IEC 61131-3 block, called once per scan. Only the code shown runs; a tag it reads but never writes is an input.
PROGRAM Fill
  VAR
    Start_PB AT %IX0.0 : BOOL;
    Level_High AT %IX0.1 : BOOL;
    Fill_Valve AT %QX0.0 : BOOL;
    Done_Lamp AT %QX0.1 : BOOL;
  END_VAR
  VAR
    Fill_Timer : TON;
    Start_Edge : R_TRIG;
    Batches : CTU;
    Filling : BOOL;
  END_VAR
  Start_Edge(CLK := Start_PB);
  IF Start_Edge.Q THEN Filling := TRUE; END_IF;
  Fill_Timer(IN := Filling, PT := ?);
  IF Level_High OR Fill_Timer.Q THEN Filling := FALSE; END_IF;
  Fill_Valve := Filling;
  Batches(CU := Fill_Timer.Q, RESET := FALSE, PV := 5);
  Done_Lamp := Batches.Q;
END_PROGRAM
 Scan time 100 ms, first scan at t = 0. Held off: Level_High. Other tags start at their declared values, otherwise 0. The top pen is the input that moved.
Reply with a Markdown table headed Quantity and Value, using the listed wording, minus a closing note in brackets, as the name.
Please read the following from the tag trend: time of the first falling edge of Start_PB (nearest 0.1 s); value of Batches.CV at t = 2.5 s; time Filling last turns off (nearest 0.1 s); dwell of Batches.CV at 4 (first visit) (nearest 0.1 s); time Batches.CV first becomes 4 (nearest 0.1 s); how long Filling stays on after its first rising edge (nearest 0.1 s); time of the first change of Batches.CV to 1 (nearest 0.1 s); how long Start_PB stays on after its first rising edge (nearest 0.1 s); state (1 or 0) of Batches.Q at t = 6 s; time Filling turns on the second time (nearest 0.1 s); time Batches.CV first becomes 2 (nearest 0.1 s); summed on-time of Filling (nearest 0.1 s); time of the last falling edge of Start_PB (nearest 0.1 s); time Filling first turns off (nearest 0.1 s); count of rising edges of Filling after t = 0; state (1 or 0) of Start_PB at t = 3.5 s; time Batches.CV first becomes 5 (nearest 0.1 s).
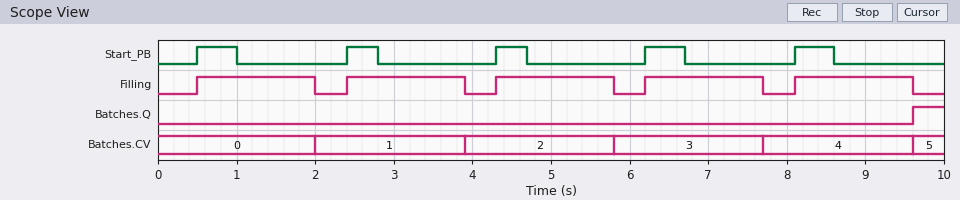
| Quantity | Value |
|---|---|
| time of the first falling edge of Start_PB | 1.0 s |
| value of Batches.CV at t = 2.5 s | 1 |
| time Filling last turns off | 9.6 s |
| dwell of Batches.CV at 4 (first visit) | 1.9 s |
| time Batches.CV first becomes 4 | 7.7 s |
| how long Filling stays on after its first rising edge | 1.5 s |
| time of the first change of Batches.CV to 1 | 2.0 s |
| how long Start_PB stays on after its first rising edge | 0.5 s |
| state (1 or 0) of Batches.Q at t = 6 s | 0 |
| time Filling turns on the second time | 2.4 s |
| time Batches.CV first becomes 2 | 3.9 s |
| summed on-time of Filling | 7.5 s |
| time of the last falling edge of Start_PB | 8.6 s |
| time Filling first turns off | 2.0 s |
| count of rising edges of Filling after t = 0 | 5 |
| state (1 or 0) of Start_PB at t = 3.5 s | 0 |
| time Batches.CV first becomes 5 | 9.6 s |
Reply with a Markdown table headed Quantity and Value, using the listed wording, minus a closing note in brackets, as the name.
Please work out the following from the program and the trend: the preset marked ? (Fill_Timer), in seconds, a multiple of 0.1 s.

| Quantity | Value |
|---|---|
| the preset marked ? (Fill_Timer), in seconds, a multiple of 0.1 s | 1.5 s |
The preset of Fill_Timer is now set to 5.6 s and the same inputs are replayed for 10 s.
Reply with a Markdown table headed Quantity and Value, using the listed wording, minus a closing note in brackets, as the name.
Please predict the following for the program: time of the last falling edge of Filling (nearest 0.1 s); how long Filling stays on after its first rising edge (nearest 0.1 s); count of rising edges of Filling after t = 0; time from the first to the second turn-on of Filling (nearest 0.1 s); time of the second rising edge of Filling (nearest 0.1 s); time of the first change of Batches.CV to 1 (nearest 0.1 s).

| Quantity | Value |
|---|---|
| time of the last falling edge of Filling | 6.1 s |
| how long Filling stays on after its first rising edge | 5.6 s |
| count of rising edges of Filling after t = 0 | 2 |
| time from the first to the second turn-on of Filling | 7.6 s |
| time of the second rising edge of Filling | 8.1 s |
| time of the first change of Batches.CV to 1 | 6.1 s |
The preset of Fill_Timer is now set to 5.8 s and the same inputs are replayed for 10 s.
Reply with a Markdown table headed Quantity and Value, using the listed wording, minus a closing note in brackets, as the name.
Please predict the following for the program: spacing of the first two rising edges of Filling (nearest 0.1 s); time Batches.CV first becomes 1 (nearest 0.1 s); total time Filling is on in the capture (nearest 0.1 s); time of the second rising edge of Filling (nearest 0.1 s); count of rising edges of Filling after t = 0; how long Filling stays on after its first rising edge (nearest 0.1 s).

| Quantity | Value |
|---|---|
| spacing of the first two rising edges of Filling | 7.6 s |
| time Batches.CV first becomes 1 | 6.3 s |
| total time Filling is on in the capture | 7.7 s |
| time of the second rising edge of Filling | 8.1 s |
| count of rising edges of Filling after t = 0 | 2 |
| how long Filling stays on after its first rising edge | 5.8 s |
